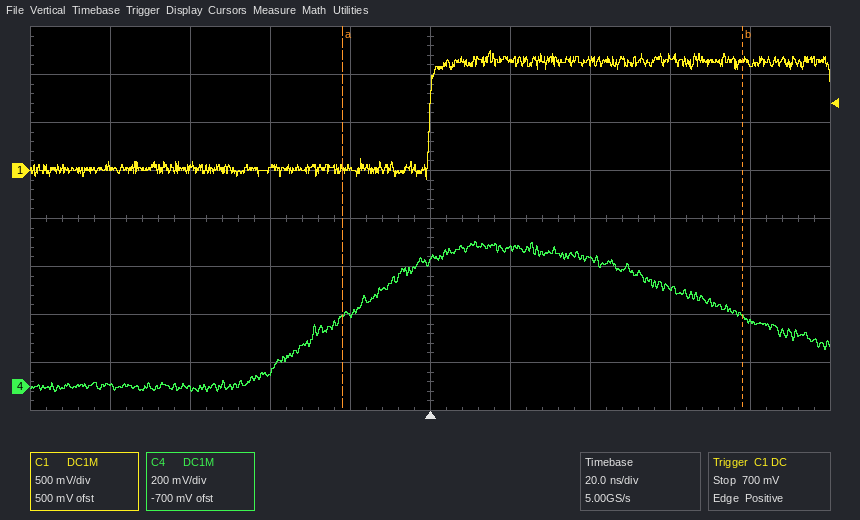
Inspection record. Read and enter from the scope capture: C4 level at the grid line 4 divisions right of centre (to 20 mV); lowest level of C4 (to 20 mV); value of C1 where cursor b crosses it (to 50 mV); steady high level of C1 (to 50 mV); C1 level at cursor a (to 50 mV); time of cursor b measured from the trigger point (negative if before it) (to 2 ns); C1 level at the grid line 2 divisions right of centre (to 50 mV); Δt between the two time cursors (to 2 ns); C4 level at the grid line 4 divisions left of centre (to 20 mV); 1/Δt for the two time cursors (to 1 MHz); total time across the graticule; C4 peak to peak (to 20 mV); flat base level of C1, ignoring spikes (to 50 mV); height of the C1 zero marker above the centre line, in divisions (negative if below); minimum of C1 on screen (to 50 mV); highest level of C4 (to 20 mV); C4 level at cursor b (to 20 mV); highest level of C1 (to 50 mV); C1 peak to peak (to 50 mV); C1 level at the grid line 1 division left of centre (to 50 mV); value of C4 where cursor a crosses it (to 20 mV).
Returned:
280 mV
-20 mV
1.15 V
1.15 V
0 mV
+78 ns
1.15 V
100 ns
0 mV
10 MHz
200 ns
620 mV
0 mV
+1.0 div
-100 mV
600 mV
300 mV
1.25 V
1.35 V
50 mV
300 mV
